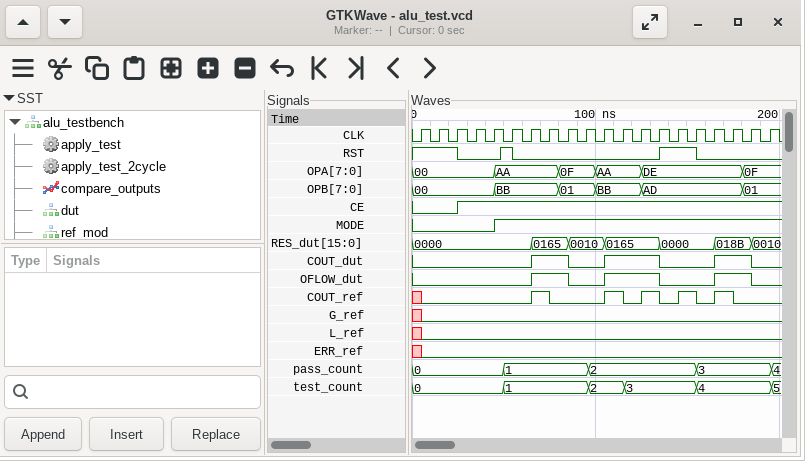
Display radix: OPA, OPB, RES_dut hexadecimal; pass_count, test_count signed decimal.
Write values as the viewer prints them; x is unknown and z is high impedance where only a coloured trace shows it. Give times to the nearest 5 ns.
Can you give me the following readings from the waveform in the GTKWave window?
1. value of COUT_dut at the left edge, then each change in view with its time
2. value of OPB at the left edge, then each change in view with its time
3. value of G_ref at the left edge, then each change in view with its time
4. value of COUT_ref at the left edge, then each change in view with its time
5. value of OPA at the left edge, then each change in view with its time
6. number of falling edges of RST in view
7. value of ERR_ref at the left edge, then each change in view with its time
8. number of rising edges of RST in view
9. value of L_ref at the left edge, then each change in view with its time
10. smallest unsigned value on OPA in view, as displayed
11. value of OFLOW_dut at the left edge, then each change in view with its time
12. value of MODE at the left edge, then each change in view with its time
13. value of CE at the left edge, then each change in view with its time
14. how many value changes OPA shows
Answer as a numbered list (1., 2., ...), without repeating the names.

1. 0, 1 at 65 ns, 0 at 85 ns, 1 at 105 ns, 0 at 135 ns, 1 at 165 ns, 0 at 185 ns
2. 00, BB at 45 ns, 01 at 80 ns, BB at 100 ns, AD at 125 ns, 01 at 180 ns
3. x, 0 at 5 ns
4. x, 0 at 5 ns, 1 at 65 ns, 0 at 75 ns, 1 at 105 ns, 0 at 115 ns, 1 at 125 ns, 0 at 135 ns, 1 at 145 ns, 0 at 155 ns, 1 at 165 ns, 0 at 175 ns
5. 00, AA at 45 ns, 0F at 80 ns, AA at 100 ns, DE at 125 ns, 0F at 180 ns
6. 3
7. x, 0 at 5 ns
8. 2
9. x, 0 at 5 ns
10. 00
11. 0, 1 at 65 ns, 0 at 85 ns, 1 at 105 ns, 0 at 135 ns, 1 at 165 ns, 0 at 185 ns
12. 0, 1 at 45 ns
13. 0, 1 at 25 ns
14. 5
